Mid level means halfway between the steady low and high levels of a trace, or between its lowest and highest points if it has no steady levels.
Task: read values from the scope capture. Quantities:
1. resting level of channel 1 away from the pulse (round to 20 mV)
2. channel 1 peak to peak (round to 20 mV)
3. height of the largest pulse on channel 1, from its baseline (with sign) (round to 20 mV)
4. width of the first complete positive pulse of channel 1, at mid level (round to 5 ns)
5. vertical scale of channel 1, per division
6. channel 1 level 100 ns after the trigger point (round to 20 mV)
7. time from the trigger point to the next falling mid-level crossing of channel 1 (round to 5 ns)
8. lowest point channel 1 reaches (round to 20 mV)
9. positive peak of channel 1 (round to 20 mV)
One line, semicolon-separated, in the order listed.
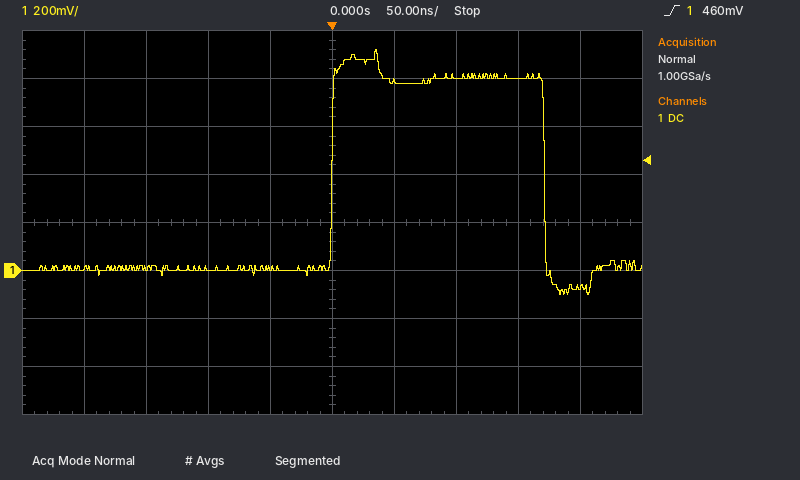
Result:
0 mV; 1.02 V; +920 mV; 170 ns; 200 mV; 800 mV; 170 ns; -100 mV; 920 mV
